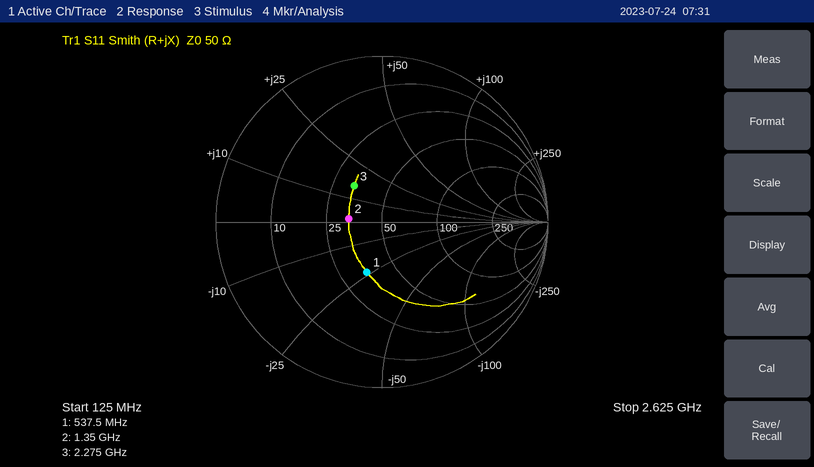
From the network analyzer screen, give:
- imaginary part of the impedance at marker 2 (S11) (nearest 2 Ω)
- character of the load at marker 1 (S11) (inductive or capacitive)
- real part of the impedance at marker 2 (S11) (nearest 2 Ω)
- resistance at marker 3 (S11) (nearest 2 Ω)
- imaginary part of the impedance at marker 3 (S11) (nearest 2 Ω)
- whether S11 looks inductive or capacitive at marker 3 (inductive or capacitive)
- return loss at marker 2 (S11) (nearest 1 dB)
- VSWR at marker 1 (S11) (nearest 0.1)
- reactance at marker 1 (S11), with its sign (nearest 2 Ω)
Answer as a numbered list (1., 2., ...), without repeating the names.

1. +2 Ω
2. capacitive
3. 34 Ω
4. 32 Ω
5. +16 Ω
6. inductive
7. 14 dB
8. 1.9
9. -24 Ω
